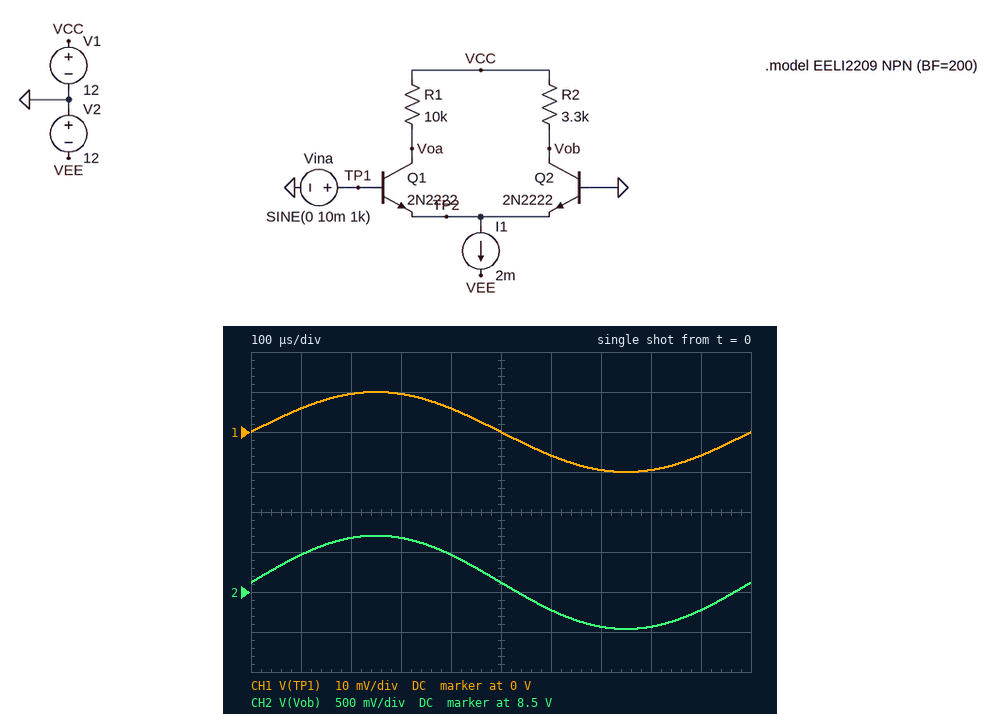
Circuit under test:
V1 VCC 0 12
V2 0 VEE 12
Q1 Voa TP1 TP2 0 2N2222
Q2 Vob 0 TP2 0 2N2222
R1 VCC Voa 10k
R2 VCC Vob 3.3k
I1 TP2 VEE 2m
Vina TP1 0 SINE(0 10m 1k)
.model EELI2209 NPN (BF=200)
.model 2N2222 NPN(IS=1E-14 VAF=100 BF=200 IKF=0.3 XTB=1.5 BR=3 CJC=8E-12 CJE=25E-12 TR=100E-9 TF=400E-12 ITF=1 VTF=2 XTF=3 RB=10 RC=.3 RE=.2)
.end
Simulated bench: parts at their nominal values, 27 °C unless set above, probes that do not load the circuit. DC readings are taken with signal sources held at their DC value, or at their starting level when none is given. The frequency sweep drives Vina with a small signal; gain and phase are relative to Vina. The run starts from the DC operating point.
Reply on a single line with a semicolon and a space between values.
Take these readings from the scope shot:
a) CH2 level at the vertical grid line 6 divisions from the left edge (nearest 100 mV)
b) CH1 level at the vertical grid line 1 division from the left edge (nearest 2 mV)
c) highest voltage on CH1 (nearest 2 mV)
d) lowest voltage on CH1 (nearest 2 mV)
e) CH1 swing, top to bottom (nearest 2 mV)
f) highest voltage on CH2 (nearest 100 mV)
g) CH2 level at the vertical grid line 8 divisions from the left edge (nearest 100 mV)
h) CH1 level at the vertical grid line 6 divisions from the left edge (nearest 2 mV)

8.3 V; 6 mV; 10 mV; -10 mV; 20 mV; 9.2 V; 8.1 V; -6 mV
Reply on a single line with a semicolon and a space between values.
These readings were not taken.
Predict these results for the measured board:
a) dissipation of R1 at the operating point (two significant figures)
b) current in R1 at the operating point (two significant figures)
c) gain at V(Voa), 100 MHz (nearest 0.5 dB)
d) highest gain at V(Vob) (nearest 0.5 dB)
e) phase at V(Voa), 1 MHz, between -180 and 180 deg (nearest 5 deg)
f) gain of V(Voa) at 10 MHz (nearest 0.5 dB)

9.3 mW; 970 µA; 13.0 dB; 35.5 dB; 160 deg; 33.0 dB
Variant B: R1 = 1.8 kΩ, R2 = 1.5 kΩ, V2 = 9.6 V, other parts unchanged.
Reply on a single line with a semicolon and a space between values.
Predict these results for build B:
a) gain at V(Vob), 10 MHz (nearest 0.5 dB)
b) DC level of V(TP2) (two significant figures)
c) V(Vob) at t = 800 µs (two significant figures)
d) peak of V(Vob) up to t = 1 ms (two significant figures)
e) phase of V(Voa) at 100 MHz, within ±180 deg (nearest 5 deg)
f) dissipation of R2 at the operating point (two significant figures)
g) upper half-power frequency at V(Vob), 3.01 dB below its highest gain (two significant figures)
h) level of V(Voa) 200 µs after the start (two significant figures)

28.0 dB; -650 mV; 10 V; 11 V; 80 deg; 1.5 mW; 22 MHz; 9.9 V
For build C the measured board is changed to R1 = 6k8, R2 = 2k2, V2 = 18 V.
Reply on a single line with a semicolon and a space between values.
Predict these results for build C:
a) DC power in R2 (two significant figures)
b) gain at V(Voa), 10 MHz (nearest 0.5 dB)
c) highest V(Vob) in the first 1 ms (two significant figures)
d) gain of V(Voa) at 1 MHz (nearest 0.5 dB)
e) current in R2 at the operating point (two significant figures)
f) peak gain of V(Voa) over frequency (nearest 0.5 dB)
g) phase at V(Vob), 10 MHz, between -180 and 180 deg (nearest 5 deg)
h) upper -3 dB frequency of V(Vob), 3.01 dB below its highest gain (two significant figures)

2.3 mW; 34.5 dB; 10 V; 41.5 dB; 1.0 mA; 42.0 dB; -35 deg; 14 MHz
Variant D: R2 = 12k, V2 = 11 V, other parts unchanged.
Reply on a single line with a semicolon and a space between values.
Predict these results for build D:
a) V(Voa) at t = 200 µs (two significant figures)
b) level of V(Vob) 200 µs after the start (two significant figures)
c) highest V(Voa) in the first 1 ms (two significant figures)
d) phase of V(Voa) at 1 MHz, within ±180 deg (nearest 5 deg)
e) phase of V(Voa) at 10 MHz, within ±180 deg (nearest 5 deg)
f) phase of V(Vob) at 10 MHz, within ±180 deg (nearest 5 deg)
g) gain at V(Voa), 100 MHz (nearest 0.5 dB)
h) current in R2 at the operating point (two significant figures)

350 mV; 2.1 V; 3.1 V; 155 deg; 100 deg; -85 deg; 12.5 dB; 990 µA
